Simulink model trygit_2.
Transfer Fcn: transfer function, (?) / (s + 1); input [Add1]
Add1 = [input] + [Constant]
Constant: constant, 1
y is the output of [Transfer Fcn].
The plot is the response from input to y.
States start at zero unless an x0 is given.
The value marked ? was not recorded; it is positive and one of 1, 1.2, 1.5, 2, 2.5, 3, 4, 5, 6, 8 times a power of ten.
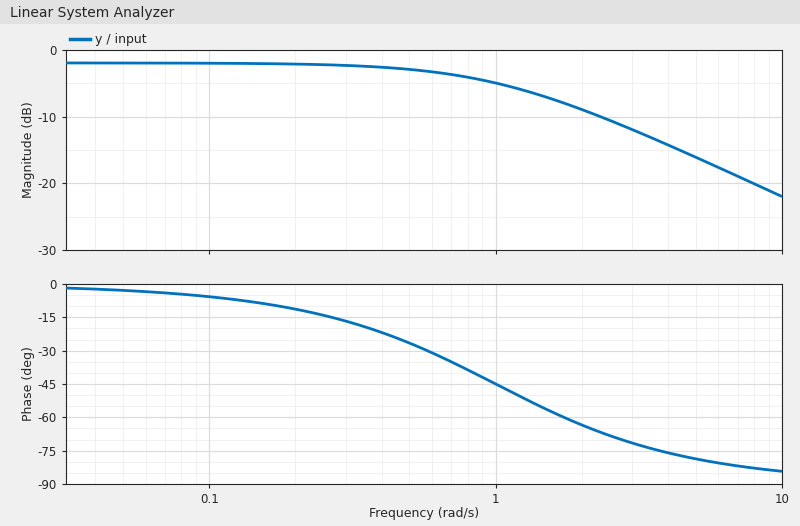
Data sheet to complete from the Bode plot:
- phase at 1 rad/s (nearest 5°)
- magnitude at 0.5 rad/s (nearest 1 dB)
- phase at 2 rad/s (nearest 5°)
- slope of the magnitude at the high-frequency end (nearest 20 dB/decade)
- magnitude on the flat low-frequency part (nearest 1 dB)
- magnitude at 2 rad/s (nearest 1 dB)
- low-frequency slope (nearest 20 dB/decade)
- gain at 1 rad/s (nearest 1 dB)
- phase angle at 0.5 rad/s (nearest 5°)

-45°
-3 dB
-65°
-20 dB/decade
-2 dB
-9 dB
0 dB/decade
-5 dB
-25°
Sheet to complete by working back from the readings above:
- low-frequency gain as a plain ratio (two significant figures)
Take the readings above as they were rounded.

0.79
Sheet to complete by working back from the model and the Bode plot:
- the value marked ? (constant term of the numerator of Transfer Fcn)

0.8
